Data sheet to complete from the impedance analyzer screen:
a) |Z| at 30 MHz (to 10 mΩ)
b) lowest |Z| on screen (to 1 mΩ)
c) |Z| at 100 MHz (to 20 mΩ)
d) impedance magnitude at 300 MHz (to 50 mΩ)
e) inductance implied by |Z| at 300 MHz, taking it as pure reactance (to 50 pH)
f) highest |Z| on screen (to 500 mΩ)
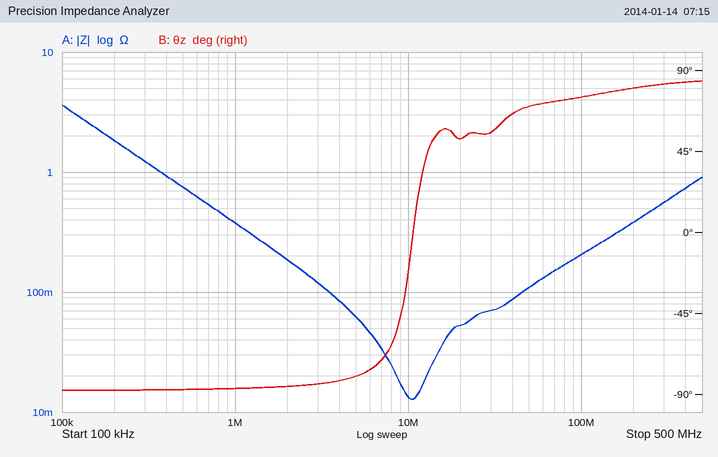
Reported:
70 mΩ
13 mΩ
200 mΩ
550 mΩ
300 pH
3.5 Ω
